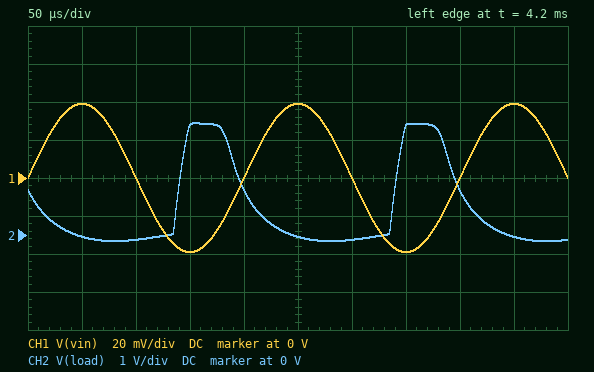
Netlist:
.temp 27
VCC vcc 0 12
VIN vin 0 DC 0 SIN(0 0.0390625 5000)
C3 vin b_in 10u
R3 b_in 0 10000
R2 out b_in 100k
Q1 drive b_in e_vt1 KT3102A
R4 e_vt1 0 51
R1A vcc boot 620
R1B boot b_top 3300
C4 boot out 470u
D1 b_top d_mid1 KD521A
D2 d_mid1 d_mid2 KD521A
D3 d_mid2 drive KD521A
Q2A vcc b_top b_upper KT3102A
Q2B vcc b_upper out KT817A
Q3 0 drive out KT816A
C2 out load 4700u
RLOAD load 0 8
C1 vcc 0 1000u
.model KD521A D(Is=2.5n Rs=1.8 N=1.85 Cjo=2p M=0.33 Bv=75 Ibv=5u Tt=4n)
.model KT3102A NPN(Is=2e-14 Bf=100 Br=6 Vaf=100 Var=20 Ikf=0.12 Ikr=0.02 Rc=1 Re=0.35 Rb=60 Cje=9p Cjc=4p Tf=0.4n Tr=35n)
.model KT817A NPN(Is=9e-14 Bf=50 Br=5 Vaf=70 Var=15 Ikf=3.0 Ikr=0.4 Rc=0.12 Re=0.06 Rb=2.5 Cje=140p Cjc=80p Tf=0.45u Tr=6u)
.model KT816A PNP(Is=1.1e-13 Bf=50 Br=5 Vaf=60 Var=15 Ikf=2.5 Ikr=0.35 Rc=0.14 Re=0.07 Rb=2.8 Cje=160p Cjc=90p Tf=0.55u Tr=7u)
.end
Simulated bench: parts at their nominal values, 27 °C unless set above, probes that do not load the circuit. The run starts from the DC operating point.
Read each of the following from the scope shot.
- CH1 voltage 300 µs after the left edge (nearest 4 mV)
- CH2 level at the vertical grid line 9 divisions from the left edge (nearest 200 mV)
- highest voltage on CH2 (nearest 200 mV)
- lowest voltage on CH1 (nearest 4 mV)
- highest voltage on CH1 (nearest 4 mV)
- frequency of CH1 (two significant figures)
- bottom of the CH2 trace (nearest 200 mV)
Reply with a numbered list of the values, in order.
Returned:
1. 0 V
2. 0 V
3. 3.0 V
4. -40 mV
5. 40 mV
6. 5.0 kHz
7. -200 mV
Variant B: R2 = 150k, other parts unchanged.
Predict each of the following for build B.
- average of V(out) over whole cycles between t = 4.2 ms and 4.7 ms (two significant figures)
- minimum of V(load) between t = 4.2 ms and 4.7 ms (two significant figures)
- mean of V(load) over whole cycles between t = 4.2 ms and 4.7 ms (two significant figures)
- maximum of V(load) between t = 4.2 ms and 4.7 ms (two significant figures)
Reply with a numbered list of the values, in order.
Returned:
1. 10 V
2. -88 mV
3. 280 mV
4. 1.1 V
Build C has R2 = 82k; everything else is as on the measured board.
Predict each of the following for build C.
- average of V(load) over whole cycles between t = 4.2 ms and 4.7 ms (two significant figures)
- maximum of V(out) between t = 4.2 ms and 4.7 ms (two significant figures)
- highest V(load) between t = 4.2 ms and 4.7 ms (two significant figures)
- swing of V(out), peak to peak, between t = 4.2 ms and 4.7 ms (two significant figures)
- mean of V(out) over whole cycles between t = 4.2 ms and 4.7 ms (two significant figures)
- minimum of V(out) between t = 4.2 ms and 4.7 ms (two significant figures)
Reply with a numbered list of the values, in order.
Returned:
1. 860 mV
2. 11 V
3. 3.8 V
4. 4.0 V
5. 8.1 V
6. 7.1 V
